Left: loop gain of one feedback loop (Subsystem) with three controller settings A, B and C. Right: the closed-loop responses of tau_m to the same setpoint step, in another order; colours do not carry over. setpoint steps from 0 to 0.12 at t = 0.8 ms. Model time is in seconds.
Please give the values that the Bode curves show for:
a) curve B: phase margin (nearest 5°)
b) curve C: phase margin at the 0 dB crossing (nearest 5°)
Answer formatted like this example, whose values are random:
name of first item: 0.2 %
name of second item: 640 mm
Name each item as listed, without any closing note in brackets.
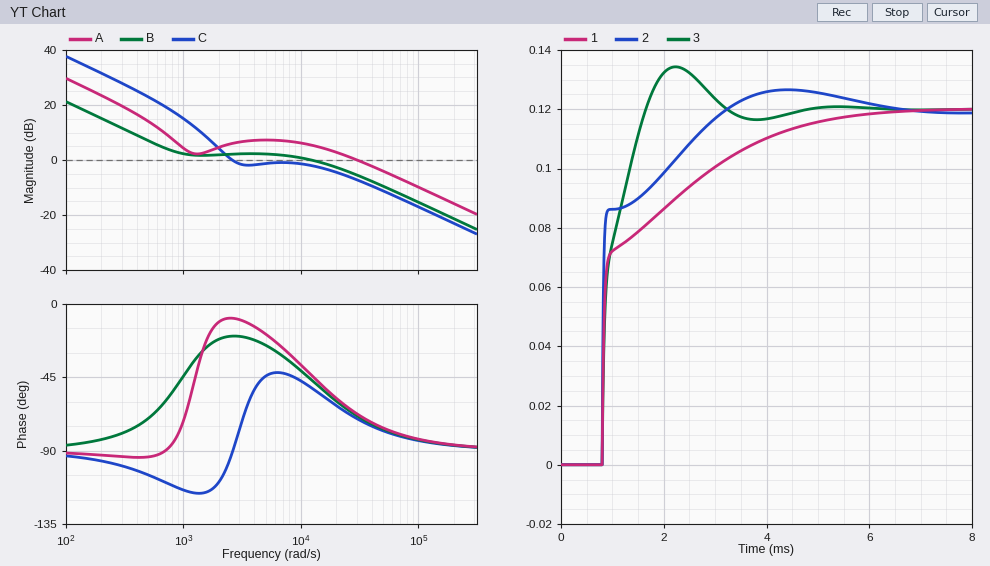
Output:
curve B: phase margin: 135°
curve C: phase margin at the 0 dB crossing: 90°
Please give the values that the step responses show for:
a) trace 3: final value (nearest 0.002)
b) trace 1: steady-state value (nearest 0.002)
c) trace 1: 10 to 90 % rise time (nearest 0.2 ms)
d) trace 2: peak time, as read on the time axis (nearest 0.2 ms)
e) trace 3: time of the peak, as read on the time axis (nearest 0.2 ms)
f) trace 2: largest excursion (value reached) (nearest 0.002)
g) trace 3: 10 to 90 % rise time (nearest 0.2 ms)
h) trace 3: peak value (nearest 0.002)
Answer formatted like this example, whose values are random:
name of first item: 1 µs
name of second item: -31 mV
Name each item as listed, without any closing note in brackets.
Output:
trace 3: final value: 0.120
trace 1: steady-state value: 0.120
trace 1: 10 to 90 % rise time: 3.0 ms
trace 2: peak time, as read on the time axis: 4.4 ms
trace 3: time of the peak, as read on the time axis: 2.2 ms
trace 2: largest excursion (value reached): 0.126
trace 3: 10 to 90 % rise time: 0.6 ms
trace 3: peak value: 0.134
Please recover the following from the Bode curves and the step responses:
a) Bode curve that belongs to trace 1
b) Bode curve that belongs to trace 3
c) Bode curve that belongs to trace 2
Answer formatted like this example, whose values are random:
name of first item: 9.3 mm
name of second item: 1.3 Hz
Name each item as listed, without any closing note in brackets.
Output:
Bode curve that belongs to trace 1: B
Bode curve that belongs to trace 3: C
Bode curve that belongs to trace 2: A
